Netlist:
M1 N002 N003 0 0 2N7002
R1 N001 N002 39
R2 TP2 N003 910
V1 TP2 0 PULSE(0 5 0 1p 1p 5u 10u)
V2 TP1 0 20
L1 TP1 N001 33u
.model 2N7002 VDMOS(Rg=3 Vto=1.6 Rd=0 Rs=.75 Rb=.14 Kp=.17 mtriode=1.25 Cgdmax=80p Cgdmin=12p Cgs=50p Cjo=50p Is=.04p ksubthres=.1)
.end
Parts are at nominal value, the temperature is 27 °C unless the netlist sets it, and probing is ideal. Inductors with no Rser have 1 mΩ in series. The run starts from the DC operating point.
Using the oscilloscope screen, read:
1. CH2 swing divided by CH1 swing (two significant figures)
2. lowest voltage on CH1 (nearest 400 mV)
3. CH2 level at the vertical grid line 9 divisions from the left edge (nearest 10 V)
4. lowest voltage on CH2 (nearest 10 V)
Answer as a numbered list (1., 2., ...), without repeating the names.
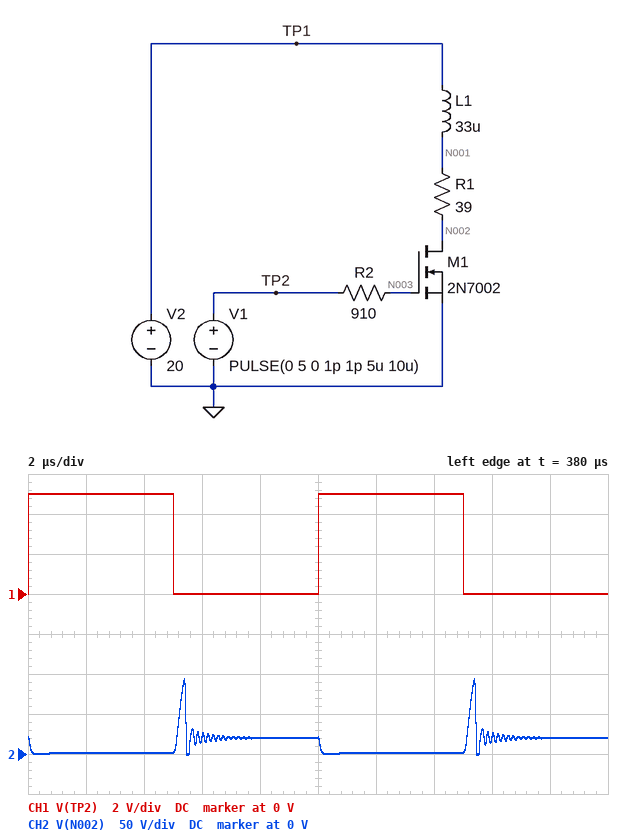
1. 19
2. 0 V
3. 20 V
4. 0 V
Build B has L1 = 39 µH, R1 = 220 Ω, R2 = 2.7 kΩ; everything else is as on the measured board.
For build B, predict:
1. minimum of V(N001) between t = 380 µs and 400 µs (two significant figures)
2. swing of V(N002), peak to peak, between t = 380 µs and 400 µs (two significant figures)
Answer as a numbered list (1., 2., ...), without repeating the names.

1. 12 V
2. 27 V
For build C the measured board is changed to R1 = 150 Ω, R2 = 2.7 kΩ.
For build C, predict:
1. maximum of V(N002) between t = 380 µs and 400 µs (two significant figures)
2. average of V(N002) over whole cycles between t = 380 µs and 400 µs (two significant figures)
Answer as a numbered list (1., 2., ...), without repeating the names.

1. 29 V
2. 9.8 V
